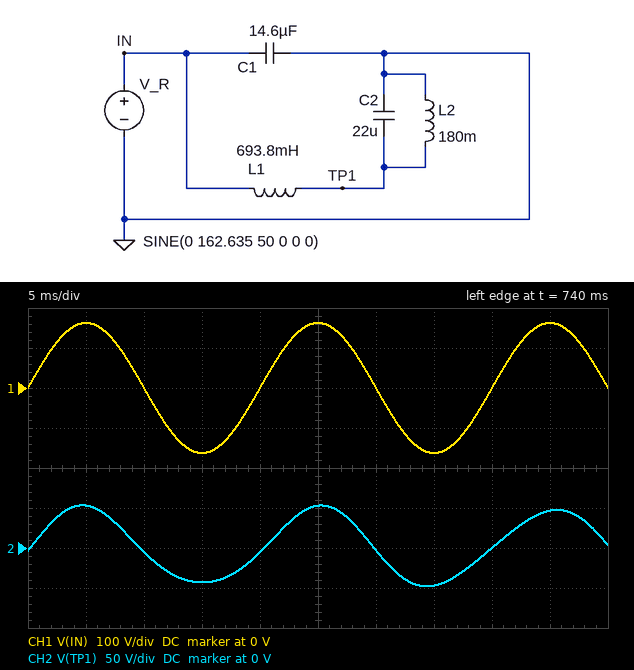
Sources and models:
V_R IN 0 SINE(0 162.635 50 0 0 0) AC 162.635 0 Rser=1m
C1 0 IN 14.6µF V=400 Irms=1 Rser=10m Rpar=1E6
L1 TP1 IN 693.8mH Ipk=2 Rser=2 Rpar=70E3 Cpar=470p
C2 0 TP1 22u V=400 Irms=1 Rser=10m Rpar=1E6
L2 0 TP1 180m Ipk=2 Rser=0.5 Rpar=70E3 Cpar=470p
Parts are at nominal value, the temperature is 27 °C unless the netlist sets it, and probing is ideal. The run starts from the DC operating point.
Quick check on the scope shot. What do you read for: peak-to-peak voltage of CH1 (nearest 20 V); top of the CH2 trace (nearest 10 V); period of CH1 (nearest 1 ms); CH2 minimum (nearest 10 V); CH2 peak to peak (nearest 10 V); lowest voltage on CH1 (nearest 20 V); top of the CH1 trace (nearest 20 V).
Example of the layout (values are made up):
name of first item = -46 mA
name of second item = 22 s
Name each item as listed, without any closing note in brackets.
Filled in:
peak-to-peak voltage of CH1 = 320 V
top of the CH2 trace = 50 V
period of CH1 = 20 ms
CH2 minimum = -50 V
CH2 peak to peak = 100 V
lowest voltage on CH1 = -160 V
top of the CH1 trace = 160 V
